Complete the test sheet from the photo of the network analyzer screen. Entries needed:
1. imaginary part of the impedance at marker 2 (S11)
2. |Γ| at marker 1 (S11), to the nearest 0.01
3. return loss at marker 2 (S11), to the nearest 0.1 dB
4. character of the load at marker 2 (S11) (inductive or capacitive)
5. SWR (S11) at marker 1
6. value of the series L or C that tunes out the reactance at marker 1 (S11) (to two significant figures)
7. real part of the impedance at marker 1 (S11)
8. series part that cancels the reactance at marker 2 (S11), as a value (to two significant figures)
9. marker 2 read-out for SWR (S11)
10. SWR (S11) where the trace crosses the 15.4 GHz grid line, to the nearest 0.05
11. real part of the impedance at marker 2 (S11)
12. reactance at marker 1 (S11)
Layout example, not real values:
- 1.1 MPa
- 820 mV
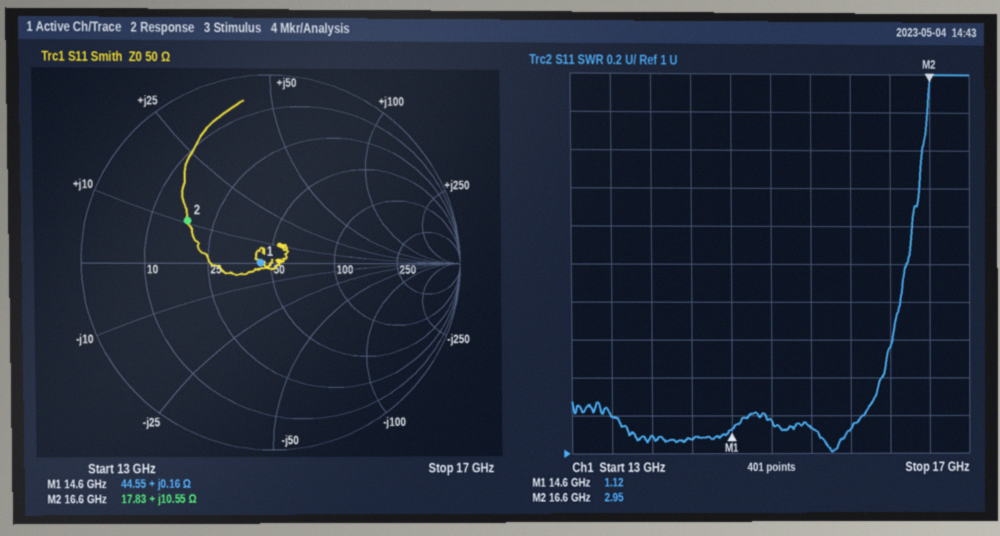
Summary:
- +10.55 Ω
- 0.06
- 6.1 dB
- inductive
- 1.12
- 68 pF
- 44.55 Ω
- 910 fF
- 2.95
- 1.15
- 17.83 Ω
- +0.16 Ω
